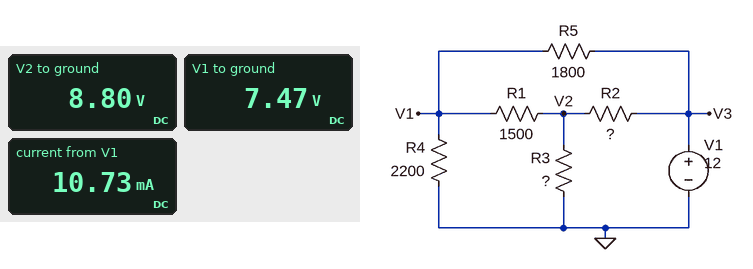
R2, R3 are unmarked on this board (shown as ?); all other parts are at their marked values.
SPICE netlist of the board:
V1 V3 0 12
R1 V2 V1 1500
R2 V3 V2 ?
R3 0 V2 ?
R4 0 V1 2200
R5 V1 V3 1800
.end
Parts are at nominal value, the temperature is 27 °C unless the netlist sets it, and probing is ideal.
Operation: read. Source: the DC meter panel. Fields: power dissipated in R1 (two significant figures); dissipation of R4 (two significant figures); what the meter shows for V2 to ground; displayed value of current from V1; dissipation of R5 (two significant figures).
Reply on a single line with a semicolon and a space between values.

1.2 mW; 25 mW; 8.80 V; 10.73 mA; 11 mW
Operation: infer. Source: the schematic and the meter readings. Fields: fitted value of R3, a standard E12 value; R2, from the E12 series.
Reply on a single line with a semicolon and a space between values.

1.2 kΩ; 390 Ω
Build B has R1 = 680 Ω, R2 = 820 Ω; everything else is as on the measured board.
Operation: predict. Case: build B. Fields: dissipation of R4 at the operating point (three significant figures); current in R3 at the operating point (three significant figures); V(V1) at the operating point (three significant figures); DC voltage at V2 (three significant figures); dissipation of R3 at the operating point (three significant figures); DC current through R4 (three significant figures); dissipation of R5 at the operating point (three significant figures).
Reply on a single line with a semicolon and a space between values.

21.3 mW; 5.84 mA; 6.84 V; 7.01 V; 40.9 mW; 3.11 mA; 14.8 mW
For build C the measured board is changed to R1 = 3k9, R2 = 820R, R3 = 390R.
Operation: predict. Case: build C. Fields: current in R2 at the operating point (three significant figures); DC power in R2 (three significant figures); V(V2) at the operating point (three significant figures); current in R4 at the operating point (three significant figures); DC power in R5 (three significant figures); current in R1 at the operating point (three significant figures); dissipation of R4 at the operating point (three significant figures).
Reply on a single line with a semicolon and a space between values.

9.75 mA; 77.9 mW; 4.01 V; 2.76 mA; 19.5 mW; 530 µA; 16.8 mW
